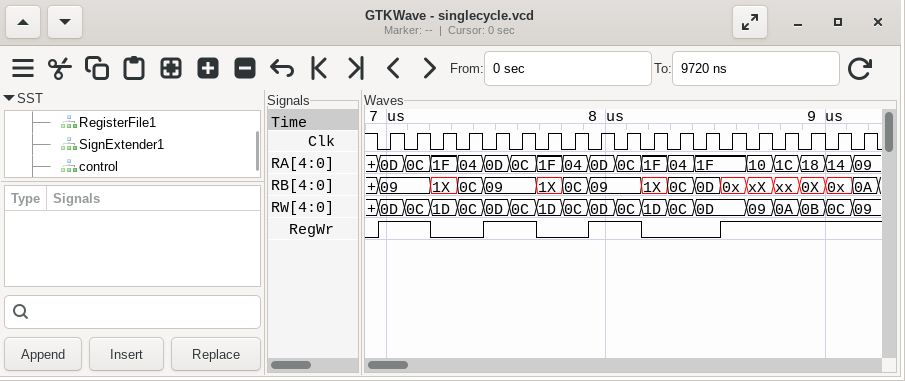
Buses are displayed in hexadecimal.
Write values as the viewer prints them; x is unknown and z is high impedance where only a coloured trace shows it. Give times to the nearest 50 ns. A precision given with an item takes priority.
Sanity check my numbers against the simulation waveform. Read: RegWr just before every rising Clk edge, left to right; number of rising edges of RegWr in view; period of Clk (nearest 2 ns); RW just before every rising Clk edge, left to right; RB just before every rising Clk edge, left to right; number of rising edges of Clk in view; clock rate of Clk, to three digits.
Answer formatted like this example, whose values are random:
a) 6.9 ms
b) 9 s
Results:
a) 1 1 0 0 1 1 0 0 1 1 0 0 0 1 1 1 1 1 1
b) 4
c) 120 ns
d) 0D, 0C, 1D, 0C, 0D, 0C, 1D, 0C, 0D, 0C, 1D, 0C, 0D, 0D, 09, 0A, 0B, 0C, 09
e) 09, 09, 1X, 0C, 09, 09, 1X, 0C, 09, 09, 1X, 0C, 0D, 0x, xX, xx, 0X, 0x, 0A
f) 19
g) 8.33 MHz
